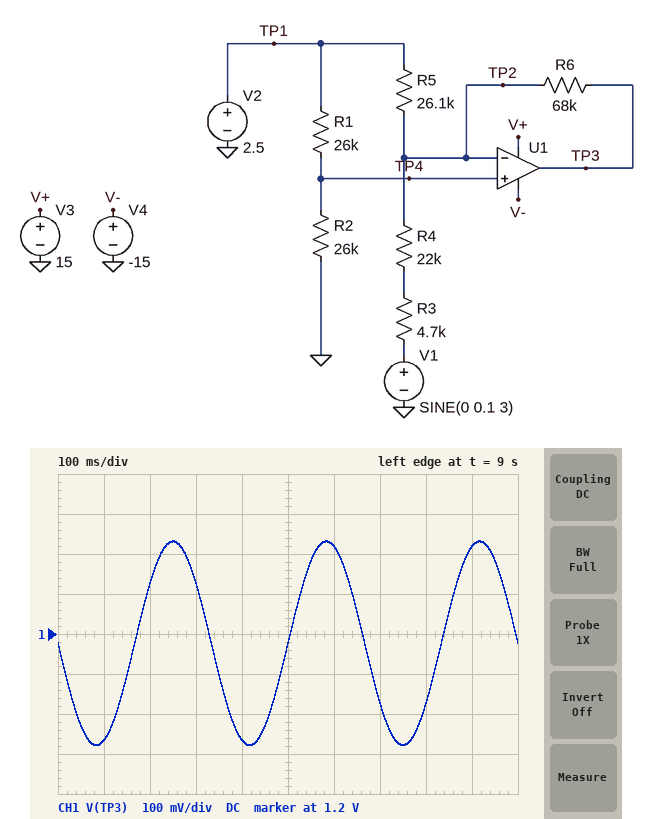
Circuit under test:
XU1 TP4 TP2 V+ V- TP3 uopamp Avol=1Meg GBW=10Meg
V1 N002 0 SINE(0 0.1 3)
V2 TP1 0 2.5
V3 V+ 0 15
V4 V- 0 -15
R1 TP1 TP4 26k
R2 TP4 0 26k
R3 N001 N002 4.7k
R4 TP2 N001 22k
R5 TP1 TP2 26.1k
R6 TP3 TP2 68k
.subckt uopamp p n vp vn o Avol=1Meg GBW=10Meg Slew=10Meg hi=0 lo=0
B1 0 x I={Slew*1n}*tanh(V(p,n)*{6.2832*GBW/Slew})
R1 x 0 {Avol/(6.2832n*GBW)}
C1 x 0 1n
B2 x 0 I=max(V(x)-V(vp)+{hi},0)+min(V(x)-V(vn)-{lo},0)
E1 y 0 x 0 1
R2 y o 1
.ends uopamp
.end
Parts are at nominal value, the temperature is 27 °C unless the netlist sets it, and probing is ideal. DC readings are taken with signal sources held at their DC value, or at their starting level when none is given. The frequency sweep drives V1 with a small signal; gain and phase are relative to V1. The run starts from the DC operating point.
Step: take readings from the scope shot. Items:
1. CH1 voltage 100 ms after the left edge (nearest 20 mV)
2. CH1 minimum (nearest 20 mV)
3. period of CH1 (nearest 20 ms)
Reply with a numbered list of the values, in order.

1. 940 mV
2. 920 mV
3. 340 ms
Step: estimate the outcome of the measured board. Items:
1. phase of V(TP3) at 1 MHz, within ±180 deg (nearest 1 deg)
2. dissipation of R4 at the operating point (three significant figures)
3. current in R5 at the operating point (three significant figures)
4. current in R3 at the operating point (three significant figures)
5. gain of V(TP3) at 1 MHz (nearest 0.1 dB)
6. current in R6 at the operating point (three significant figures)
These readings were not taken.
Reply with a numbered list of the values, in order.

1. 148 deg
2. 48.2 µW
3. 47.9 µA
4. 46.8 µA
5. 6.7 dB
6. 1.08 µA
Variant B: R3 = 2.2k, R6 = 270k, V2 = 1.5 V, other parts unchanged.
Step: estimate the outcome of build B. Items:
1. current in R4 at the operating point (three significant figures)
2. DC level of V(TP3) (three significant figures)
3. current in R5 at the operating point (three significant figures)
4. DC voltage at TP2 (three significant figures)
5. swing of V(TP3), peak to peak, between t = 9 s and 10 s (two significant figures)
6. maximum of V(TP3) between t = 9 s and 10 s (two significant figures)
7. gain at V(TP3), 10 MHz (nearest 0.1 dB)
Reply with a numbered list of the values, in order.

1. 31.0 µA
2. 1.36 V
3. 28.7 µA
4. 750 mV
5. 2.2 V
6. 2.5 V
7. -6.1 dB
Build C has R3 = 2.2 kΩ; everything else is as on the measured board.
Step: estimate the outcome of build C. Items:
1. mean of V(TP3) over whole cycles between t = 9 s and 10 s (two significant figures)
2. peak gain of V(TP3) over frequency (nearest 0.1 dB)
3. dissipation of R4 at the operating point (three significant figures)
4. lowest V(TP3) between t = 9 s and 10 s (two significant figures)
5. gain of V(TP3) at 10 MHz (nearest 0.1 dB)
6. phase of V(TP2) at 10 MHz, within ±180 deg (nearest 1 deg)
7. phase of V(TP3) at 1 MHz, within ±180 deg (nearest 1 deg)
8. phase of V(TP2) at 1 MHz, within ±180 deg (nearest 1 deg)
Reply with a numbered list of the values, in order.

1. 1.5 V
2. 9.0 dB
3. 58.7 µW
4. 1.2 V
5. -7.3 dB
6. 9 deg
7. 147 deg
8. 57 deg
